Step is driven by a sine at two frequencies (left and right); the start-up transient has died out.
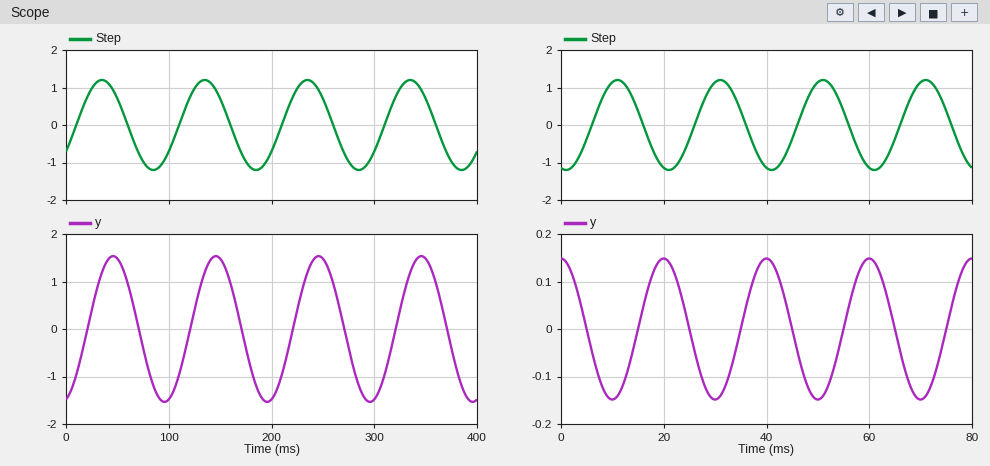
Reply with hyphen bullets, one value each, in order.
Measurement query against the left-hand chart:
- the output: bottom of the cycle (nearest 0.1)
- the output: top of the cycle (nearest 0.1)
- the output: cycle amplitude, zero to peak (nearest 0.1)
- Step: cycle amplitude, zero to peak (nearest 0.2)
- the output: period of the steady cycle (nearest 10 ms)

- -1.5
- 1.5
- 1.5
- 1.2
- 100 ms
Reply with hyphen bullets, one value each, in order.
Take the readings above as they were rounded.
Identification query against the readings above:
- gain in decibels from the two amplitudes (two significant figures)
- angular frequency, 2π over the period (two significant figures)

- 1.9 dB
- 0.063 rad/ms
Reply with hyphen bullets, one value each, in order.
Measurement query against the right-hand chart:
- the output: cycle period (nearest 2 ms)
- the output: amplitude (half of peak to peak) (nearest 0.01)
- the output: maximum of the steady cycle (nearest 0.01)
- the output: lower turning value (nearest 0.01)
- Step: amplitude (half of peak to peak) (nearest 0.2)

- 20 ms
- 0.15
- 0.15
- -0.15
- 1.2
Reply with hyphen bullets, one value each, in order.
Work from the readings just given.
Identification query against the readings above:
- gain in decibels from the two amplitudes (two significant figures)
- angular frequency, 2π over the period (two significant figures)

- -18 dB
- 0.31 rad/ms
